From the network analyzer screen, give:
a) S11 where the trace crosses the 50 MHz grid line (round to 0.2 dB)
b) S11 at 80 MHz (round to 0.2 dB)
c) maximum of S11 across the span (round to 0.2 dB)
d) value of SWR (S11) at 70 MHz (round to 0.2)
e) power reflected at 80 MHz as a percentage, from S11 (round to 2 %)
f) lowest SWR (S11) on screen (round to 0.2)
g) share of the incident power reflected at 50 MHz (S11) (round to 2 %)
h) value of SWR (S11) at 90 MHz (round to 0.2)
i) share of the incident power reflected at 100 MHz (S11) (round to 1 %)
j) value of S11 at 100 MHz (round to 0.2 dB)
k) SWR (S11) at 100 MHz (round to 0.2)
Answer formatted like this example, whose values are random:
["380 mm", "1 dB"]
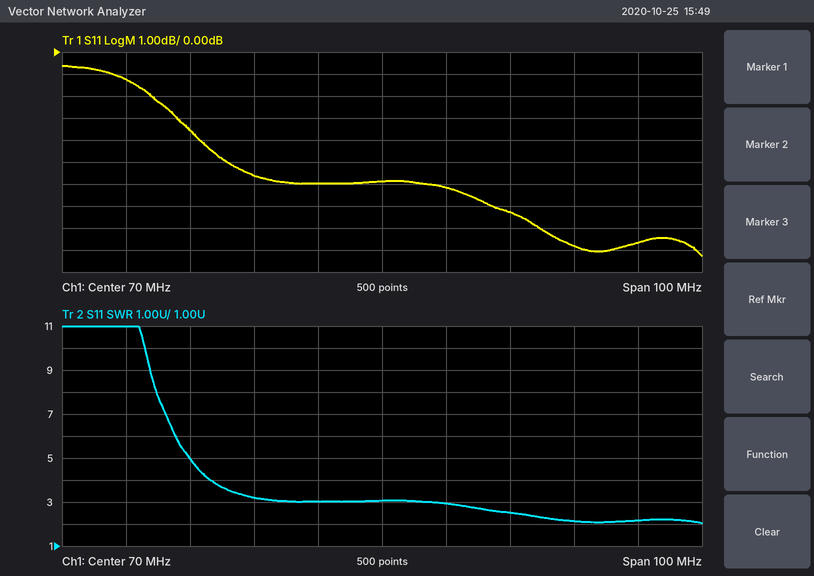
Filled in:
["-5.6 dB", "-6.2 dB", "-0.6 dB", "3.0", "24 %", "2.0", "28 %", "2.6", "13 %", "-8.8 dB", "2.2"]
